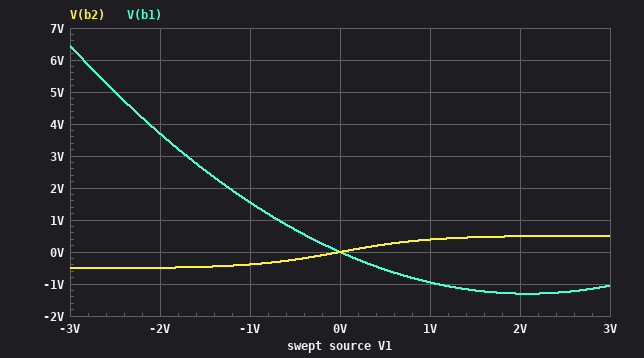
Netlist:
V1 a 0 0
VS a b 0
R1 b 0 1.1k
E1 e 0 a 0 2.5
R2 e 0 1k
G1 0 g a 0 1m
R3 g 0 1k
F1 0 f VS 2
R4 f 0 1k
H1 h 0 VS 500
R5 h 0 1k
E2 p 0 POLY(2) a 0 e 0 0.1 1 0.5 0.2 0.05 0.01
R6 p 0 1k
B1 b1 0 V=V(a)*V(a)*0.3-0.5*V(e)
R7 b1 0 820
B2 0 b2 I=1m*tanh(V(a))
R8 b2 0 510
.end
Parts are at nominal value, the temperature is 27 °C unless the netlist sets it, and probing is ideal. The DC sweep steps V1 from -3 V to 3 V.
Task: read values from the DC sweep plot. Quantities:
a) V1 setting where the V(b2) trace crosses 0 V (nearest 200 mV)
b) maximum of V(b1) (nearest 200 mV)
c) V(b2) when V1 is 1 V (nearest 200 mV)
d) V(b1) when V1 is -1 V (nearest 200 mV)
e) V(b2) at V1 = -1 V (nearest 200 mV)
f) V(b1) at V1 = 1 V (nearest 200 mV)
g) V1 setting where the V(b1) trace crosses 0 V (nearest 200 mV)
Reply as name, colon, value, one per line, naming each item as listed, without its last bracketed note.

V1 setting where the V(b2) trace crosses 0 V: 0 V
maximum of V(b1): 6.4 V
V(b2) when V1 is 1 V: 400 mV
V(b1) when V1 is -1 V: 1.6 V
V(b2) at V1 = -1 V: -400 mV
V(b1) at V1 = 1 V: -1.0 V
V1 setting where the V(b1) trace crosses 0 V: 0 V
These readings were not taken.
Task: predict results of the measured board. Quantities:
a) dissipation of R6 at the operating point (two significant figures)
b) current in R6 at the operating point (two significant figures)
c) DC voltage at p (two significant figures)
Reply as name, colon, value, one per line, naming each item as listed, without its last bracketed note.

dissipation of R6 at the operating point: 10 µW
current in R6 at the operating point: 100 µA
DC voltage at p: 100 mV
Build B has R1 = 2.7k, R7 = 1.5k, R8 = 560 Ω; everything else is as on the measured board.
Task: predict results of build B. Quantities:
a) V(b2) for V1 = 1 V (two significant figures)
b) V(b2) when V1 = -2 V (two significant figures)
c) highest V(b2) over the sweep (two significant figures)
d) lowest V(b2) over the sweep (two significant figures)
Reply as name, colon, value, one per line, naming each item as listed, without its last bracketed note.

V(b2) for V1 = 1 V: 430 mV
V(b2) when V1 = -2 V: -540 mV
highest V(b2) over the sweep: 560 mV
lowest V(b2) over the sweep: -560 mV
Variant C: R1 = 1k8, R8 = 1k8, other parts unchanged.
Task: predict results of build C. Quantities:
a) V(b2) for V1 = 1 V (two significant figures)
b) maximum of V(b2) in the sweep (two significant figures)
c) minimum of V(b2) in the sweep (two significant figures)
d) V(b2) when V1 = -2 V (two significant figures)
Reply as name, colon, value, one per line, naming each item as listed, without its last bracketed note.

V(b2) for V1 = 1 V: 1.4 V
maximum of V(b2) in the sweep: 1.8 V
minimum of V(b2) in the sweep: -1.8 V
V(b2) when V1 = -2 V: -1.7 V
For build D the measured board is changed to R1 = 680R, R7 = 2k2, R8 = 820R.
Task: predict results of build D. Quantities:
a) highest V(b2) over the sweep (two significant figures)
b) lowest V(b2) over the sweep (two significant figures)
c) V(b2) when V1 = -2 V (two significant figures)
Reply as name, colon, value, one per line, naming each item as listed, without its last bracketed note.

highest V(b2) over the sweep: 820 mV
lowest V(b2) over the sweep: -820 mV
V(b2) when V1 = -2 V: -790 mV
